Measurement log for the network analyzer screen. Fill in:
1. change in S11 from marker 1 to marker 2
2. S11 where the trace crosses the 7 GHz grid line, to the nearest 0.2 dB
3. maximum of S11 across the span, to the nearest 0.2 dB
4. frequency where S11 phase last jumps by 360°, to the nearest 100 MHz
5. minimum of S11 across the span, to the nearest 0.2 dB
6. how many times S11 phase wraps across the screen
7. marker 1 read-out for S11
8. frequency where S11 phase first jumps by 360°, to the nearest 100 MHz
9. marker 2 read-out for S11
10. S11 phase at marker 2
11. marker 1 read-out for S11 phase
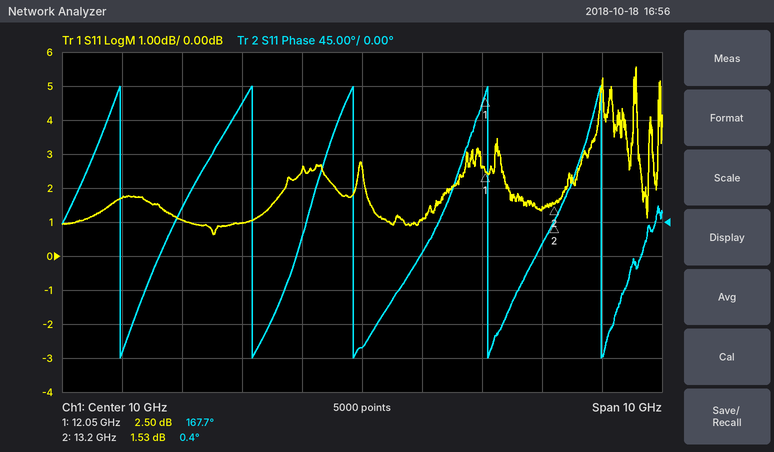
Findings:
-0.97 dB
1.0 dB
5.6 dB
14.0 GHz
0.6 dB
5
2.50 dB
6.0 GHz
1.53 dB
0.4°
167.7°
